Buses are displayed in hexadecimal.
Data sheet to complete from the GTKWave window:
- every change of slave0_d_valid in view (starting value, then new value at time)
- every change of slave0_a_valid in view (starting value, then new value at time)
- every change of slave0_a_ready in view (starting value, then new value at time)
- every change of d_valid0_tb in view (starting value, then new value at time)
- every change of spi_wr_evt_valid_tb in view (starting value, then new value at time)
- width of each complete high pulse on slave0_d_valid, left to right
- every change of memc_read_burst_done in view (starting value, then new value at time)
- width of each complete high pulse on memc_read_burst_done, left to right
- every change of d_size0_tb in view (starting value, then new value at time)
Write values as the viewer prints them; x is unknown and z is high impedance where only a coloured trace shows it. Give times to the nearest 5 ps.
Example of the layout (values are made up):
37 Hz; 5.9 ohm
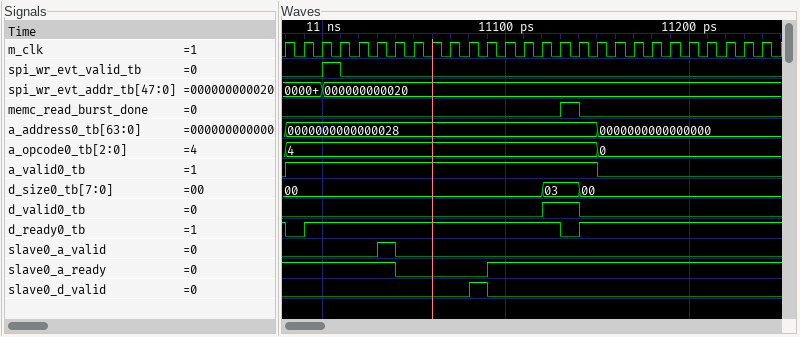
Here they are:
0, 1 at 11080 ps, 0 at 11090 ps; 0, 1 at 11030 ps, 0 at 11040 ps; 1, 0 at 11040 ps, 1 at 11090 ps; 0, 1 at 11120 ps, 0 at 11140 ps; 0, 1 at 11000 ps, 0 at 11010 ps; 10 ps; 0, 1 at 11130 ps, 0 at 11140 ps; 10 ps; 00, 03 at 11120 ps, 00 at 11140 ps
